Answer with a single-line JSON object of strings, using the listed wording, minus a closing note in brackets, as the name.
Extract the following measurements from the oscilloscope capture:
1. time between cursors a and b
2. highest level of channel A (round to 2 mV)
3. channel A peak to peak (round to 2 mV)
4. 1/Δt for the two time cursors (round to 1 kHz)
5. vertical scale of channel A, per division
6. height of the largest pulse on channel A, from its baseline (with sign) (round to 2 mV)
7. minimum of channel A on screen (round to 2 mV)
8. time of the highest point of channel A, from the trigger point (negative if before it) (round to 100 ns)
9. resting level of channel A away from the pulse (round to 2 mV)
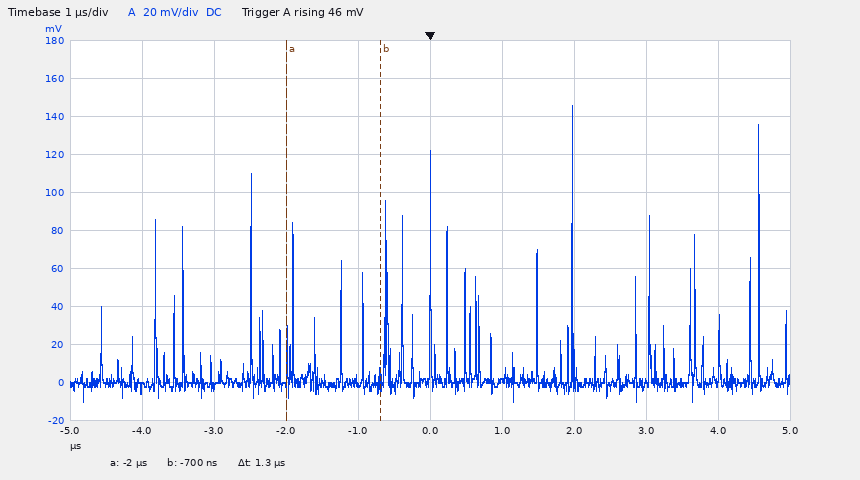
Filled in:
{"time between cursors a and b": "1.3 µs", "highest level of channel A": "146 mV", "channel A peak to peak": "156 mV", "1/Δt for the two time cursors": "769 kHz", "vertical scale of channel A, per division": "20 mV", "height of the largest pulse on channel A, from its baseline (with sign)": "+146 mV", "minimum of channel A on screen": "-10 mV", "time of the highest point of channel A, from the trigger point (negative if before it)": "+2.0 µs", "resting level of channel A away from the pulse": "0 mV"}
